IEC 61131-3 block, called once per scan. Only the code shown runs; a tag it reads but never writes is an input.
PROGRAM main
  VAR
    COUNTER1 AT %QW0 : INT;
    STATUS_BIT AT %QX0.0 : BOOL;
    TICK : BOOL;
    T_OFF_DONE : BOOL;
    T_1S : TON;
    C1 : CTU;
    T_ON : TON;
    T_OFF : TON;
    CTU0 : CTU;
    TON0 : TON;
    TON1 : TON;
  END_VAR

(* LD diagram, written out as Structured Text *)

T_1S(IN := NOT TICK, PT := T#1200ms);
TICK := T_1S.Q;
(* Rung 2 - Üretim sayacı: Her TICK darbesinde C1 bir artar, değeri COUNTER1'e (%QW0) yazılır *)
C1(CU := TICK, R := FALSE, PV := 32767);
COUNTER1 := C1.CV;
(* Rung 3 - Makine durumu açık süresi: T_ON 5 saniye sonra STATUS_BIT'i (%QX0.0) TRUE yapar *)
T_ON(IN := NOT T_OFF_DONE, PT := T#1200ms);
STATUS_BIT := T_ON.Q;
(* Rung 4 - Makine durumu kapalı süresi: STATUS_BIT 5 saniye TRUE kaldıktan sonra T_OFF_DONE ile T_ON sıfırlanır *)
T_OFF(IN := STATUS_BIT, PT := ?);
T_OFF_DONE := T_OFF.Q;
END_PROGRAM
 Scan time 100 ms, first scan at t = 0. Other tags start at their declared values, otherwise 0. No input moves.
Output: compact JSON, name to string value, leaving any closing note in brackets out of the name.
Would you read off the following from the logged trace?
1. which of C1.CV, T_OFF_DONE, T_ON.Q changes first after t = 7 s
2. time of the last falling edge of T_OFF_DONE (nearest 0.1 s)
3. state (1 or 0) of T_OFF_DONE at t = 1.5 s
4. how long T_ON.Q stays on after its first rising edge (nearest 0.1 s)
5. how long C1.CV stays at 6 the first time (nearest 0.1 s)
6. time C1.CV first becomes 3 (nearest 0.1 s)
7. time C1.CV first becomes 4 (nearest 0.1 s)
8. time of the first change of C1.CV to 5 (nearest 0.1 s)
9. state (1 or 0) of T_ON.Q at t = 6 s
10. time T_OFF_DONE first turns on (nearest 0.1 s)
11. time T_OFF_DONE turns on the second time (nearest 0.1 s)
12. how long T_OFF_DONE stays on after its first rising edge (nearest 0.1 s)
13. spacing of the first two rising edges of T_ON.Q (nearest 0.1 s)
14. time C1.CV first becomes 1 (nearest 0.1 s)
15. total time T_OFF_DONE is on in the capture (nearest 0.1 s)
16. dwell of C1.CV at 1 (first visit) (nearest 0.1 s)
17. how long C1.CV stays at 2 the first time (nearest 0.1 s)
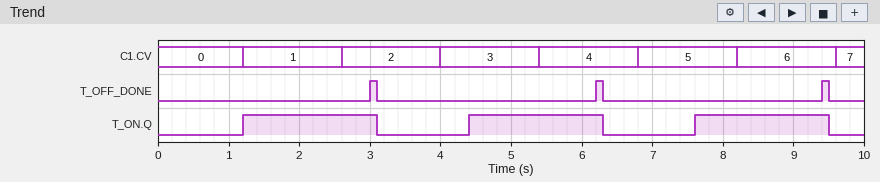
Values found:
{"which of C1.CV, T_OFF_DONE, T_ON.Q changes first after t = 7 s": "T_ON.Q", "time of the last falling edge of T_OFF_DONE": "9.5 s", "state (1 or 0) of T_OFF_DONE at t = 1.5 s": "0", "how long T_ON.Q stays on after its first rising edge": "1.9 s", "how long C1.CV stays at 6 the first time": "1.4 s", "time C1.CV first becomes 3": "4.0 s", "time C1.CV first becomes 4": "5.4 s", "time of the first change of C1.CV to 5": "6.8 s", "state (1 or 0) of T_ON.Q at t = 6 s": "1", "time T_OFF_DONE first turns on": "3.0 s", "time T_OFF_DONE turns on the second time": "6.2 s", "how long T_OFF_DONE stays on after its first rising edge": "0.1 s", "spacing of the first two rising edges of T_ON.Q": "3.2 s", "time C1.CV first becomes 1": "1.2 s", "total time T_OFF_DONE is on in the capture": "0.3 s", "dwell of C1.CV at 1 (first visit)": "1.4 s", "how long C1.CV stays at 2 the first time": "1.4 s"}
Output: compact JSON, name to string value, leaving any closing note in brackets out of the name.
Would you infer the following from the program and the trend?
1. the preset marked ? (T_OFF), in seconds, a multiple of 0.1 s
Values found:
{"the preset marked ? (T_OFF), in seconds, a multiple of 0.1 s": "1.8 s"}
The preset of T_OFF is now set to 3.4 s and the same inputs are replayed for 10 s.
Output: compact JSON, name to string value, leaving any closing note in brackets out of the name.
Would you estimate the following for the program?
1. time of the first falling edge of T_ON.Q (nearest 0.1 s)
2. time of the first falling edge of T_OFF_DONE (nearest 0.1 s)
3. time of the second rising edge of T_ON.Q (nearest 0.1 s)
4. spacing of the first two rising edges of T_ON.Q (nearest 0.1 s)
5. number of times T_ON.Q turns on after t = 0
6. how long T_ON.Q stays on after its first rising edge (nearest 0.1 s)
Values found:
{"time of the first falling edge of T_ON.Q": "4.7 s", "time of the first falling edge of T_OFF_DONE": "4.7 s", "time of the second rising edge of T_ON.Q": "6.0 s", "spacing of the first two rising edges of T_ON.Q": "4.8 s", "number of times T_ON.Q turns on after t = 0": "2", "how long T_ON.Q stays on after its first rising edge": "3.5 s"}
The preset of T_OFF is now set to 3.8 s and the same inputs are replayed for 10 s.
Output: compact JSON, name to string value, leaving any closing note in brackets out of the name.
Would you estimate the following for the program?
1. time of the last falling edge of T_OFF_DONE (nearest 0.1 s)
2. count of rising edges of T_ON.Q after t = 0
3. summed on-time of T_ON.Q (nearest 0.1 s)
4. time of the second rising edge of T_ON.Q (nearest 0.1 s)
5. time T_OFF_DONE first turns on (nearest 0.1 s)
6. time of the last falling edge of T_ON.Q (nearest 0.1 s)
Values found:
{"time of the last falling edge of T_OFF_DONE": "5.1 s", "count of rising edges of T_ON.Q after t = 0": "2", "summed on-time of T_ON.Q": "7.5 s", "time of the second rising edge of T_ON.Q": "6.4 s", "time T_OFF_DONE first turns on": "5.0 s", "time of the last falling edge of T_ON.Q": "5.1 s"}
